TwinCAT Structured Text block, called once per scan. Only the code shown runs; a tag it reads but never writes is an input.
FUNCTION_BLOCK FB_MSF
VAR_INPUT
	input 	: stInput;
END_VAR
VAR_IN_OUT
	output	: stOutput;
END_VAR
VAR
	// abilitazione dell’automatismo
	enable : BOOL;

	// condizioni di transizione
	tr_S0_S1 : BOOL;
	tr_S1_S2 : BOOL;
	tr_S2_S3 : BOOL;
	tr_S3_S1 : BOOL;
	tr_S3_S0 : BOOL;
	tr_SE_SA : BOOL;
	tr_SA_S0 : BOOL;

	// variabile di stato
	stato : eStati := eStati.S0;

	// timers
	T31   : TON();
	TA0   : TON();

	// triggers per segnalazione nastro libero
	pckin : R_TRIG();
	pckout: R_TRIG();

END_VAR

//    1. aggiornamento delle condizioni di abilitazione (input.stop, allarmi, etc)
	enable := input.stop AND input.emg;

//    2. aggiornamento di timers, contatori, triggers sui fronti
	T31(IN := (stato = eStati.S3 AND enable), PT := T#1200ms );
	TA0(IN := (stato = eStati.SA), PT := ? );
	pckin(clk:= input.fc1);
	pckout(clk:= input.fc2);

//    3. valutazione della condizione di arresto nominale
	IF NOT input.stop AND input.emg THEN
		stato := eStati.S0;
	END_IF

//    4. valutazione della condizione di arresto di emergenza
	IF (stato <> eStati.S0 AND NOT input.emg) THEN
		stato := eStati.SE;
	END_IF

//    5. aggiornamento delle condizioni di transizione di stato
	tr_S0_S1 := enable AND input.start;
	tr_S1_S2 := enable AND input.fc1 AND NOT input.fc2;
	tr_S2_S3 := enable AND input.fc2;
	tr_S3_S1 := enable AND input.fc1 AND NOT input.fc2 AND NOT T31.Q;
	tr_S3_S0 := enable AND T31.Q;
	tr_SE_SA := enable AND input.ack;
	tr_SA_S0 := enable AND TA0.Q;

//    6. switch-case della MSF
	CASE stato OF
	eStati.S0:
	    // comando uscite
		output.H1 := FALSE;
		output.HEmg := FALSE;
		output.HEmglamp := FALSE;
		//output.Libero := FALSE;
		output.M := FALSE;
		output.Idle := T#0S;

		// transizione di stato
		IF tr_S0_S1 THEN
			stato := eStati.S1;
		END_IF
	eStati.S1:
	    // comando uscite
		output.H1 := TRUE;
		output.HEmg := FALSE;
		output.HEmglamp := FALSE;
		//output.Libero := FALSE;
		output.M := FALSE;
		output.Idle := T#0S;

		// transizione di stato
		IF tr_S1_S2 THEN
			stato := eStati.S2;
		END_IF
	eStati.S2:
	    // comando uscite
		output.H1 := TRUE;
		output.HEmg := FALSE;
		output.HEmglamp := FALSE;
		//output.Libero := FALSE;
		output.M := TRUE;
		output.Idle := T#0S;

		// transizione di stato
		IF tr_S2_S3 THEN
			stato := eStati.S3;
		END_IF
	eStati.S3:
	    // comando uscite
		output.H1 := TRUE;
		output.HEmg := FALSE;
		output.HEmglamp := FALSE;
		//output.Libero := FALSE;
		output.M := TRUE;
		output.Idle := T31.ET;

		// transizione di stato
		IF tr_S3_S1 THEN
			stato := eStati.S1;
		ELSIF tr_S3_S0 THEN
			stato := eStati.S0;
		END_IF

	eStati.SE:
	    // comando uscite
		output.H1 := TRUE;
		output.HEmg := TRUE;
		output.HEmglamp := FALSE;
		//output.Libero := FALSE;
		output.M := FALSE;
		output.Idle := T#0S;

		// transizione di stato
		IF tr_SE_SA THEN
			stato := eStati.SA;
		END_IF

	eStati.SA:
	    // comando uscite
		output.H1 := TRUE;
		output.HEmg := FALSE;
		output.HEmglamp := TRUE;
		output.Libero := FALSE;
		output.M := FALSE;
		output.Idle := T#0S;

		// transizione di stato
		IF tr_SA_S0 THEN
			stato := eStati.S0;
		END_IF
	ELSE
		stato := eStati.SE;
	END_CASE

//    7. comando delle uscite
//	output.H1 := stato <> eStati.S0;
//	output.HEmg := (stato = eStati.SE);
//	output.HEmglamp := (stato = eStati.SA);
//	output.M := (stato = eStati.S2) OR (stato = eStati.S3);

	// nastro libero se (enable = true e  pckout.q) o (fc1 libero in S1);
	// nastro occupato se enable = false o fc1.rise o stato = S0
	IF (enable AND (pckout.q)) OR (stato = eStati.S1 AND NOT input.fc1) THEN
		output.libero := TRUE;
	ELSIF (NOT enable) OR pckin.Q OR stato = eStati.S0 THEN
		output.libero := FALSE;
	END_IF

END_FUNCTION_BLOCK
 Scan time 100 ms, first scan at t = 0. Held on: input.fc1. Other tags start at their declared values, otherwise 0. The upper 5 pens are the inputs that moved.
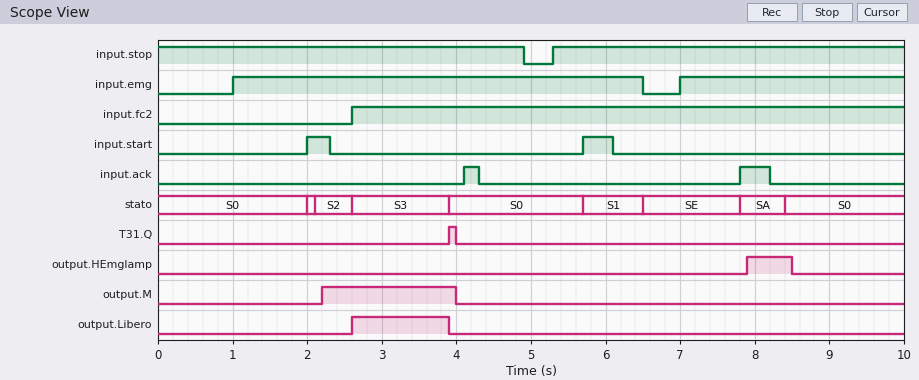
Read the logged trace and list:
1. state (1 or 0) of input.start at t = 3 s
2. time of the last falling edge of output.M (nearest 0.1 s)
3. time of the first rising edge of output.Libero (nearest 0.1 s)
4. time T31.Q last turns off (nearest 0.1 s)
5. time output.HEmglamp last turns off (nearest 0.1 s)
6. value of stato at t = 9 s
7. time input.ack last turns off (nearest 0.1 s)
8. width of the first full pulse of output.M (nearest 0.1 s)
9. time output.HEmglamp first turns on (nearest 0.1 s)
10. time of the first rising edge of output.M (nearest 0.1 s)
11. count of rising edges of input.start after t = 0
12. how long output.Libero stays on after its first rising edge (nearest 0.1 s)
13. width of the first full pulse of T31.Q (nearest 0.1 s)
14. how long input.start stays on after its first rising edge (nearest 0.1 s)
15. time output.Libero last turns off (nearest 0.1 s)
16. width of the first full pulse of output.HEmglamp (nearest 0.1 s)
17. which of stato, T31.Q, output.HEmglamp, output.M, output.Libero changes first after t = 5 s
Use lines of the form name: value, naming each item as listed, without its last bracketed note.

state (1 or 0) of input.start at t = 3 s: 0
time of the last falling edge of output.M: 4.0 s
time of the first rising edge of output.Libero: 2.6 s
time T31.Q last turns off: 4.0 s
time output.HEmglamp last turns off: 8.5 s
value of stato at t = 9 s: S0
time input.ack last turns off: 8.2 s
width of the first full pulse of output.M: 1.8 s
time output.HEmglamp first turns on: 7.9 s
time of the first rising edge of output.M: 2.2 s
count of rising edges of input.start after t = 0: 2
how long output.Libero stays on after its first rising edge: 1.3 s
width of the first full pulse of T31.Q: 0.1 s
how long input.start stays on after its first rising edge: 0.3 s
time output.Libero last turns off: 3.9 s
width of the first full pulse of output.HEmglamp: 0.6 s
which of stato, T31.Q, output.HEmglamp, output.M, output.Libero changes first after t = 5 s: stato
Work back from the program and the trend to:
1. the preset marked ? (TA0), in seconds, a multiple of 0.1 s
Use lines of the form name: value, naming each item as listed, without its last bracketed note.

the preset marked ? (TA0), in seconds, a multiple of 0.1 s: 0.5 s
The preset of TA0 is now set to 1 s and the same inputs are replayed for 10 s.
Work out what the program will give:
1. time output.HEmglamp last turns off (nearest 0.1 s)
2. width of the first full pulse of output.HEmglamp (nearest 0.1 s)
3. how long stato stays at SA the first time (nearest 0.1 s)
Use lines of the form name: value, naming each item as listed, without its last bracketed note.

time output.HEmglamp last turns off: 9.0 s
width of the first full pulse of output.HEmglamp: 1.1 s
how long stato stays at SA the first time: 1.1 s
